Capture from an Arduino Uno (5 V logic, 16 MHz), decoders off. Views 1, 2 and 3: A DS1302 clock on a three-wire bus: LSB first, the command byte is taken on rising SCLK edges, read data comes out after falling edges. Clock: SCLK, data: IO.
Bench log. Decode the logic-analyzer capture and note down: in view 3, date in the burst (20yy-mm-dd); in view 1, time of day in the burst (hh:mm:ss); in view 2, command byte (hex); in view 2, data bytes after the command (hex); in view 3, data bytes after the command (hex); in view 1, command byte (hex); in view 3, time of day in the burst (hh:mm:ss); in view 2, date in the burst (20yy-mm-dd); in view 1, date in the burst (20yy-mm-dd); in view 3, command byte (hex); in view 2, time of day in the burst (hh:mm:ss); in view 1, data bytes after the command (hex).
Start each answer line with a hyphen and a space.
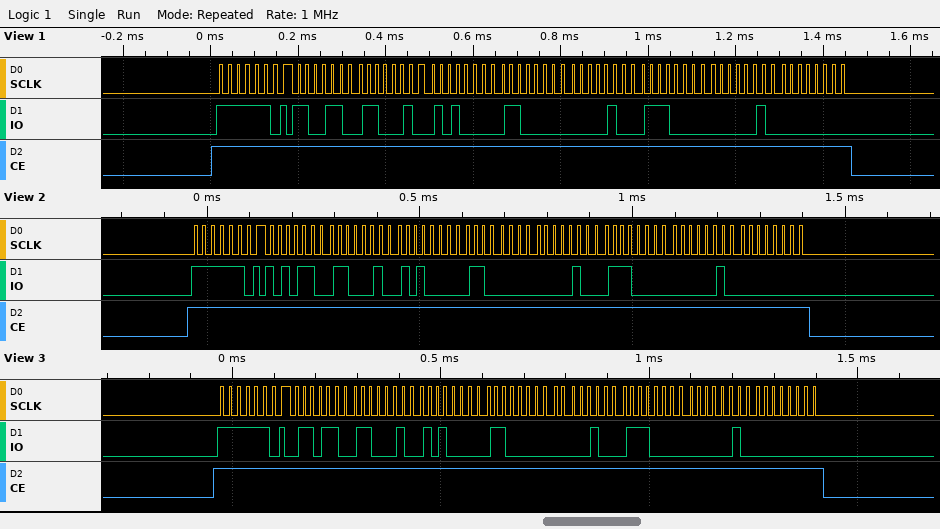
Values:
- 2020-10-03
- 05:23:33
- 0xBF
- 35 23 05 03 10 07 20 00
- 36 23 05 03 10 07 20 00
- 0xBF
- 05:23:36
- 2020-10-03
- 2020-10-03
- 0xBF
- 05:23:35
- 33 23 05 03 10 07 20 00
